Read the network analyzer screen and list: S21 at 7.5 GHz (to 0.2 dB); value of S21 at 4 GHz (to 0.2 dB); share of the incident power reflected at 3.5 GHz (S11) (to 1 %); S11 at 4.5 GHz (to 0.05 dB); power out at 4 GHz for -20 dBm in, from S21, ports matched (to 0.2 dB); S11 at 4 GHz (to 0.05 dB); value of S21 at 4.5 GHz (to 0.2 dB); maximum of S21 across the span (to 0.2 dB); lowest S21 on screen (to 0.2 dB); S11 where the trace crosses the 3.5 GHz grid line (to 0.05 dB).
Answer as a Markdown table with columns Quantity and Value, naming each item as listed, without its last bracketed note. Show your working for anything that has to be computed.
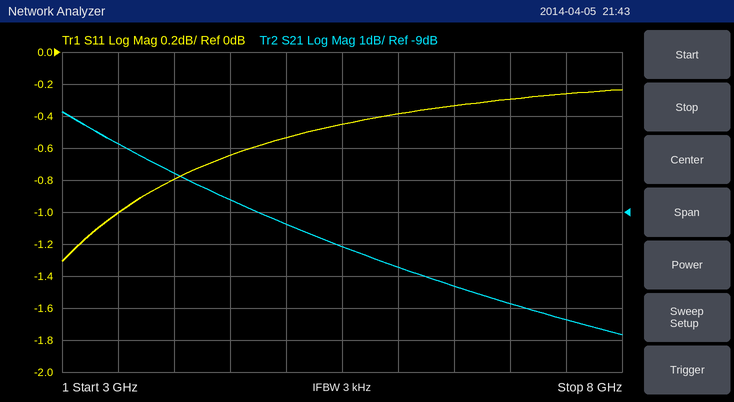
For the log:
| Quantity | Value |
|---|---|
| S21 at 7.5 GHz | -12.4 dB |
| value of S21 at 4 GHz | -7.8 dB |
| share of the incident power reflected at 3.5 GHz (S11) | 10^(-1/10) ≈ 79 % |
| S11 at 4.5 GHz | -0.65 dB |
| power out at 4 GHz for -20 dBm in, from S21, ports matched | -20 dBm + (-7.8 dB) = -27.8 dBm |
| S11 at 4 GHz | -0.80 dB |
| value of S21 at 4.5 GHz | -8.6 dB |
| maximum of S21 across the span | -5.8 dB |
| lowest S21 on screen | -12.8 dB |
| S11 where the trace crosses the 3.5 GHz grid line | -1.00 dB |
